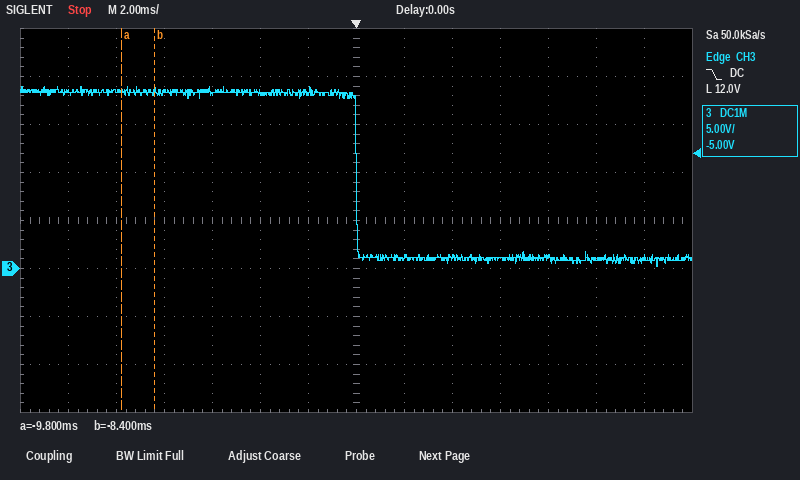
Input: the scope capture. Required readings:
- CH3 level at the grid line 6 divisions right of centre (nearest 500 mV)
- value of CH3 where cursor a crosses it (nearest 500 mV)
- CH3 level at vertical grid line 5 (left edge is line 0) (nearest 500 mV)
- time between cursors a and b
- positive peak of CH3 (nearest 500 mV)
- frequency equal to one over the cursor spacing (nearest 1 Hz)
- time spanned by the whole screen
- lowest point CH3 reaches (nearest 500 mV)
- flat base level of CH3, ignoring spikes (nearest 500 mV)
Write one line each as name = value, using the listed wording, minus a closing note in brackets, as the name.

CH3 level at the grid line 6 divisions right of centre = 1.0 V
value of CH3 where cursor a crosses it = 18.5 V
CH3 level at vertical grid line 5 (left edge is line 0) = 18.5 V
time between cursors a and b = 1.4 ms
positive peak of CH3 = 19.0 V
frequency equal to one over the cursor spacing = 714 Hz
time spanned by the whole screen = 28 ms
lowest point CH3 reaches = 0.0 V
flat base level of CH3, ignoring spikes = 1.0 V
